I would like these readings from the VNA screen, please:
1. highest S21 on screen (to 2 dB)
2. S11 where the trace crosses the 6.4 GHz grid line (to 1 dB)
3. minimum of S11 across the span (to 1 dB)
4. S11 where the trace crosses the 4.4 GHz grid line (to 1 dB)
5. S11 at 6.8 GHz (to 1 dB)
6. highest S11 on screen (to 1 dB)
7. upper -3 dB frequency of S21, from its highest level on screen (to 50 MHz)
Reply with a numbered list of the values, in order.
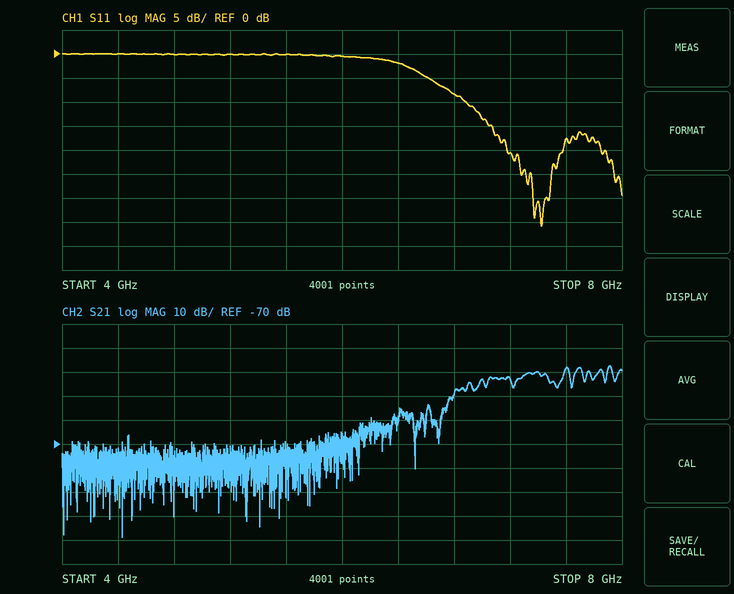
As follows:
1. -38 dB
2. -2 dB
3. -36 dB
4. 0 dB
5. -8 dB
6. 0 dB
7. 7.95 GHz
